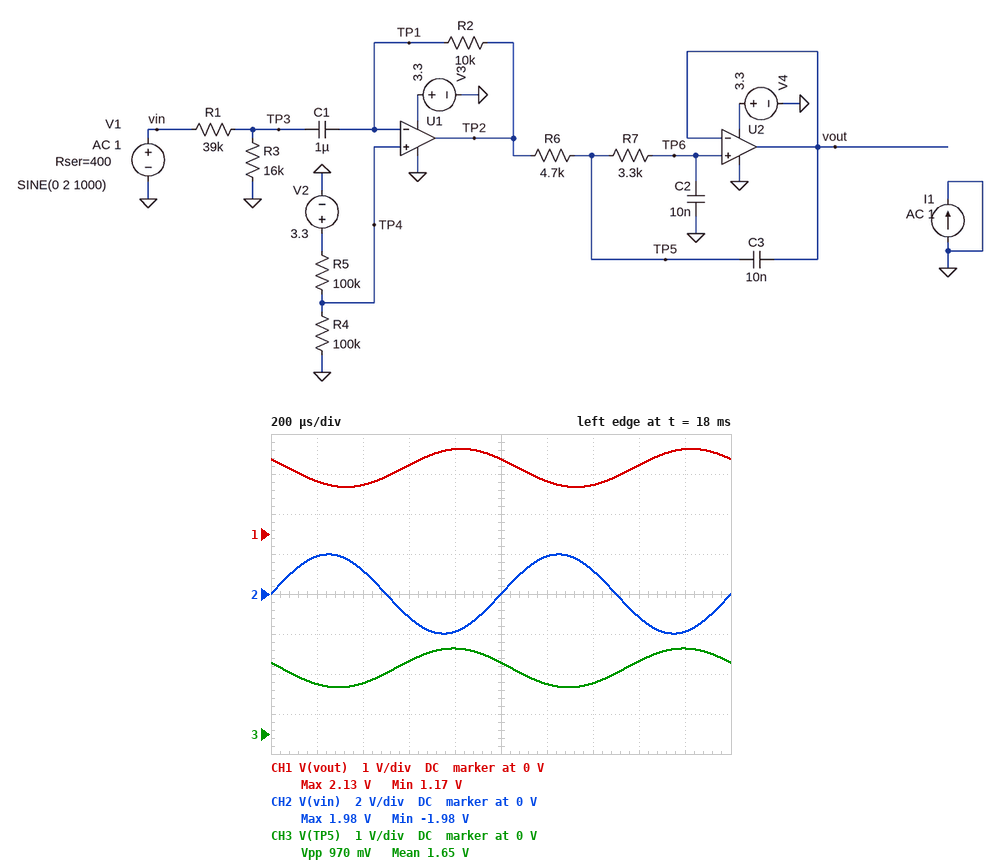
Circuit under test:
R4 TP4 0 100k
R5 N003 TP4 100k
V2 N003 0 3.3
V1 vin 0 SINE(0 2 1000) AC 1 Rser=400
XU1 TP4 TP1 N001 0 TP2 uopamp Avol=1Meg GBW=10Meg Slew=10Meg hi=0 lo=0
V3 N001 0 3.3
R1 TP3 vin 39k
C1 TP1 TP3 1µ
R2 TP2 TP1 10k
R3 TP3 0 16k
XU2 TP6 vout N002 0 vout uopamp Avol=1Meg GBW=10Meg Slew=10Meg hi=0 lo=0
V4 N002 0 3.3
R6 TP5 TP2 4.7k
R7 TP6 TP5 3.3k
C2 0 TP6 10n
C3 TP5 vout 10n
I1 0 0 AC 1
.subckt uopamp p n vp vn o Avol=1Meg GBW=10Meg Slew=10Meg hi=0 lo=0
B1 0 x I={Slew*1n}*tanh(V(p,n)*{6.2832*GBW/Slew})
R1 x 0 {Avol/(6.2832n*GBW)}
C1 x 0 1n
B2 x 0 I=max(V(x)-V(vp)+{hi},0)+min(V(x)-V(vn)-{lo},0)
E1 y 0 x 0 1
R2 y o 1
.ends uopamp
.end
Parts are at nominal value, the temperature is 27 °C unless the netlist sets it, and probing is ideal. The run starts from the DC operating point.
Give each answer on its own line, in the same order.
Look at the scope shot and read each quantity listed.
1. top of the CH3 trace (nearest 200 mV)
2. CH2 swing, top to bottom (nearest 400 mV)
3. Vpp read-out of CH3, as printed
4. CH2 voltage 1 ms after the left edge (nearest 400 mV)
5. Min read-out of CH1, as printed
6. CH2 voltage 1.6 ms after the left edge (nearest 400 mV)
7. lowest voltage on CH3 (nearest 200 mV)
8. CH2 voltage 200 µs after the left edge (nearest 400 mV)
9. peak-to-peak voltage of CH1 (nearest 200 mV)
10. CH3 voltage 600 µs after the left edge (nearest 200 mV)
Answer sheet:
2.2 V
4.0 V
970 mV
0 V
1.17 V
-1.2 V
1.2 V
2.0 V
1.0 V
1.8 V
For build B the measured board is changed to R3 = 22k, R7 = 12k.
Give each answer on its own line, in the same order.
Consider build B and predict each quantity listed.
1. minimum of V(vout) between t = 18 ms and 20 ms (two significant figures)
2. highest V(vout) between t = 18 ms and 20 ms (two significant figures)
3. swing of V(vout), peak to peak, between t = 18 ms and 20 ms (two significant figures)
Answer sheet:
1.3 V
2.0 V
780 mV
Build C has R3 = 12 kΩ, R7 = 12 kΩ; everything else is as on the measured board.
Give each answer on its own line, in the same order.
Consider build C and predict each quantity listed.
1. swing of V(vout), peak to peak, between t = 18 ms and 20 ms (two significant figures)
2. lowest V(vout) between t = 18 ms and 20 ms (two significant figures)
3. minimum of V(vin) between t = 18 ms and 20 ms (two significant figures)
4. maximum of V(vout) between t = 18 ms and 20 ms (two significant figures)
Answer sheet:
780 mV
1.3 V
-2.0 V
2.0 V
